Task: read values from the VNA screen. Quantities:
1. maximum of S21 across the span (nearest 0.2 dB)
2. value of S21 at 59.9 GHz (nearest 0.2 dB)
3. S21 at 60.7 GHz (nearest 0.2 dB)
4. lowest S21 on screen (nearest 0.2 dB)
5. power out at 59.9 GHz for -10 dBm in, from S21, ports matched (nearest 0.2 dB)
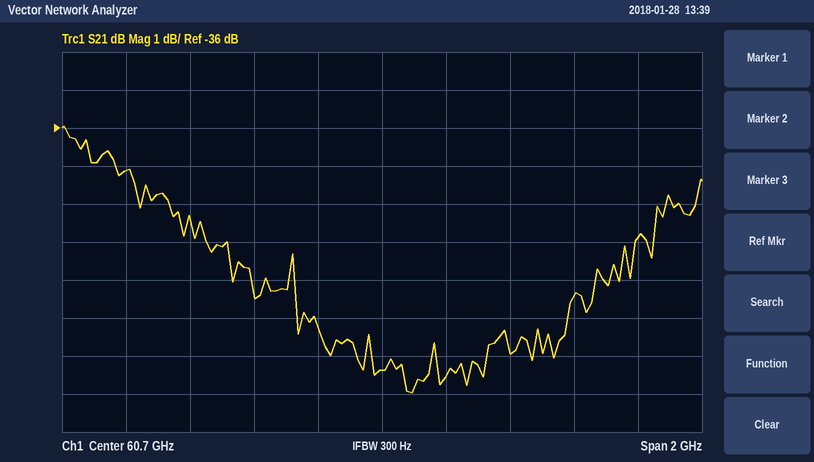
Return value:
-36.0 dB
-37.2 dB
-42.4 dB
-43.0 dB
-47.2 dBm
